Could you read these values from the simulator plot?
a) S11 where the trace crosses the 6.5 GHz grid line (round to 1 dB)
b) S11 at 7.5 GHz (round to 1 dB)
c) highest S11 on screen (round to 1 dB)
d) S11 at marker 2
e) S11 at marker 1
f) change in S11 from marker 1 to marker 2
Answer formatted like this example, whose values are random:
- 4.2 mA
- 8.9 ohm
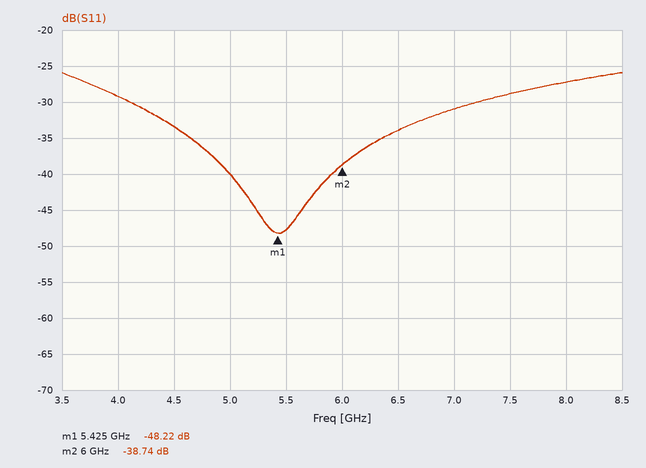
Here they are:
- -34 dB
- -29 dB
- -26 dB
- -38.74 dB
- -48.22 dB
- 9.48 dB
